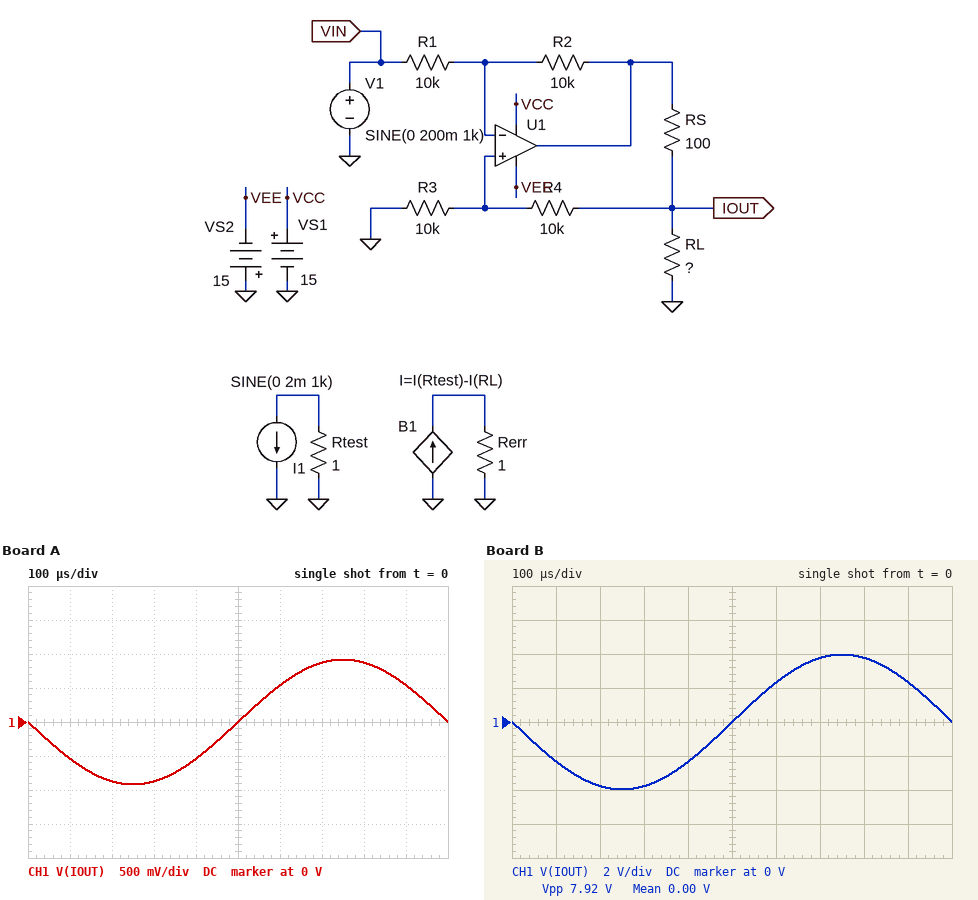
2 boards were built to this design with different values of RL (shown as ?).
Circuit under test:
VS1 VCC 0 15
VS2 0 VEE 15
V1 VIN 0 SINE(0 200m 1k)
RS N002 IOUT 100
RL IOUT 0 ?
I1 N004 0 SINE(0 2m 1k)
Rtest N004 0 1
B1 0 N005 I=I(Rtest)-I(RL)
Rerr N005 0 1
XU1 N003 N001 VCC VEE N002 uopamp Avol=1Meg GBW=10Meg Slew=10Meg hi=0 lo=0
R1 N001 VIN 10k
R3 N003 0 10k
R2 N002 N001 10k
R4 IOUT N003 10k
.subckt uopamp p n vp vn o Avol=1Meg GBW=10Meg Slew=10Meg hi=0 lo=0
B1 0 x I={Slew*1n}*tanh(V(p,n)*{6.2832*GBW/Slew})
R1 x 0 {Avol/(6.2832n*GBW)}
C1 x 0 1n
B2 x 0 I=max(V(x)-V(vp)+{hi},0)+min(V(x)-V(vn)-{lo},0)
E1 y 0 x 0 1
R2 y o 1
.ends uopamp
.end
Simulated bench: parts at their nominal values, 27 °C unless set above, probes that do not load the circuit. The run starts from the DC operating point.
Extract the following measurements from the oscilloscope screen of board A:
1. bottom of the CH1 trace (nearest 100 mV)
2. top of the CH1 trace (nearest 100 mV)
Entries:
-900 mV
900 mV
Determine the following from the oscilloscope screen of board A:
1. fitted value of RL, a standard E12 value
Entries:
470 Ω
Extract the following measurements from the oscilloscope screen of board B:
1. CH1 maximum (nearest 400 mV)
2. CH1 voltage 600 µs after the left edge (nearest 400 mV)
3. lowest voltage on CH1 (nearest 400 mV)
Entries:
4.0 V
2.4 V
-4.0 V
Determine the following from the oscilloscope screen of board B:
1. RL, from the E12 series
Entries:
2.2 kΩ
